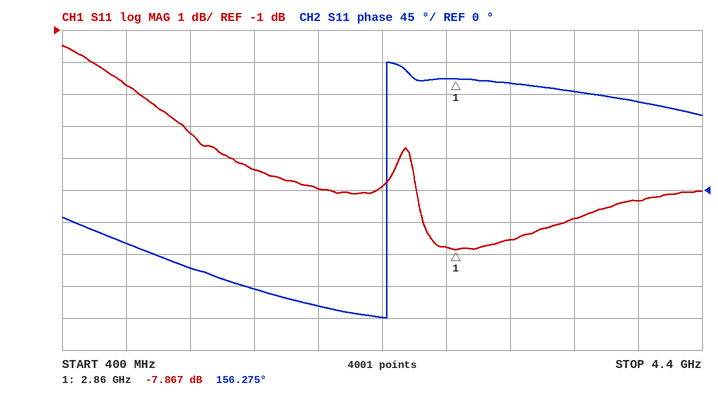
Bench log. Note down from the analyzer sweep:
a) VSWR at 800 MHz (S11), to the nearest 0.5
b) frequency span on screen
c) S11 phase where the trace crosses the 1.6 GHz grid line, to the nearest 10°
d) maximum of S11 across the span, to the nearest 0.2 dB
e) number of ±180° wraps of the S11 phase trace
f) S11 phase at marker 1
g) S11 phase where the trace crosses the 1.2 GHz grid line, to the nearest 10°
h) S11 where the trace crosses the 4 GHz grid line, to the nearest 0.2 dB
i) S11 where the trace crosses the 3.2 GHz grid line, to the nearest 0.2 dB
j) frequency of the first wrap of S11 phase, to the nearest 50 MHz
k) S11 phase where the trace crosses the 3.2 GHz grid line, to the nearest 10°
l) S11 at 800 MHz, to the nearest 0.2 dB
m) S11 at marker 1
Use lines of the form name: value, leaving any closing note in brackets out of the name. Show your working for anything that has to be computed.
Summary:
VSWR at 800 MHz (S11), to the nearest 0.5: |Γ| = 10^(-2.8/20) = 0.7244; VSWR = (1 + 0.7244)/(1 − 0.7244) ≈ 6.26, so 6.5 to the nearest 0.5
frequency span on screen: 4 GHz
S11 phase where the trace crosses the 1.6 GHz grid line, to the nearest 10°: -140°
maximum of S11 across the span, to the nearest 0.2 dB: -1.4 dB
number of ±180° wraps of the S11 phase trace: 1
S11 phase at marker 1: 156.275°
S11 phase where the trace crosses the 1.2 GHz grid line, to the nearest 10°: -110°
S11 where the trace crosses the 4 GHz grid line, to the nearest 0.2 dB: -6.4 dB
S11 where the trace crosses the 3.2 GHz grid line, to the nearest 0.2 dB: -7.6 dB
frequency of the first wrap of S11 phase, to the nearest 50 MHz: 2.45 GHz
S11 phase where the trace crosses the 3.2 GHz grid line, to the nearest 10°: 150°
S11 at 800 MHz, to the nearest 0.2 dB: -2.8 dB
S11 at marker 1: -7.867 dB
